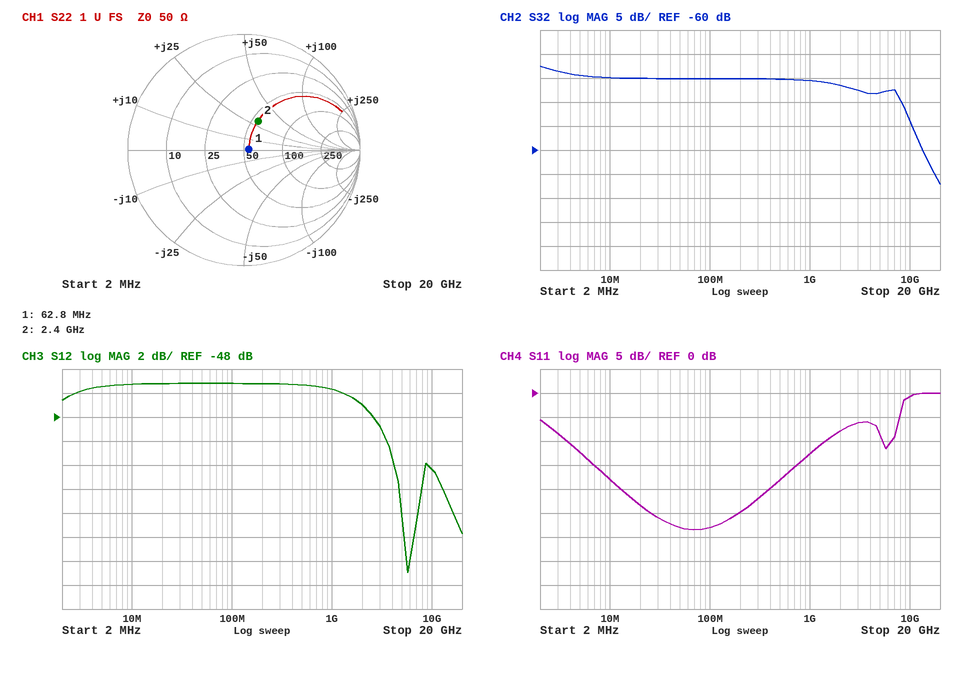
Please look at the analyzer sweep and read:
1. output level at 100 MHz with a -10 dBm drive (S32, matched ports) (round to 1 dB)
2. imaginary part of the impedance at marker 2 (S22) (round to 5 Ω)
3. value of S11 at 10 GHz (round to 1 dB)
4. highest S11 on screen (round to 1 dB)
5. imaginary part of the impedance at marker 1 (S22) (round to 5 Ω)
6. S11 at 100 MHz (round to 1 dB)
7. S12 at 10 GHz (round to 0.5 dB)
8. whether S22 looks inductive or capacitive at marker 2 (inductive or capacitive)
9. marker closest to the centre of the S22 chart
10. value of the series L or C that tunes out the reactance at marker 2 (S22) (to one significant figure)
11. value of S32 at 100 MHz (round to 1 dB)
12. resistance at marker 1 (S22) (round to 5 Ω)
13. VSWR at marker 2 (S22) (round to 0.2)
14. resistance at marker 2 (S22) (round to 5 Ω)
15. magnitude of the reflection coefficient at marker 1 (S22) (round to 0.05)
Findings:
-55 dBm
+30 Ω
-1 dB
0 dB
0 Ω
-28 dB
-52.5 dB
inductive
marker 1
2 pF
-45 dB
55 Ω
1.8
55 Ω
0.05
